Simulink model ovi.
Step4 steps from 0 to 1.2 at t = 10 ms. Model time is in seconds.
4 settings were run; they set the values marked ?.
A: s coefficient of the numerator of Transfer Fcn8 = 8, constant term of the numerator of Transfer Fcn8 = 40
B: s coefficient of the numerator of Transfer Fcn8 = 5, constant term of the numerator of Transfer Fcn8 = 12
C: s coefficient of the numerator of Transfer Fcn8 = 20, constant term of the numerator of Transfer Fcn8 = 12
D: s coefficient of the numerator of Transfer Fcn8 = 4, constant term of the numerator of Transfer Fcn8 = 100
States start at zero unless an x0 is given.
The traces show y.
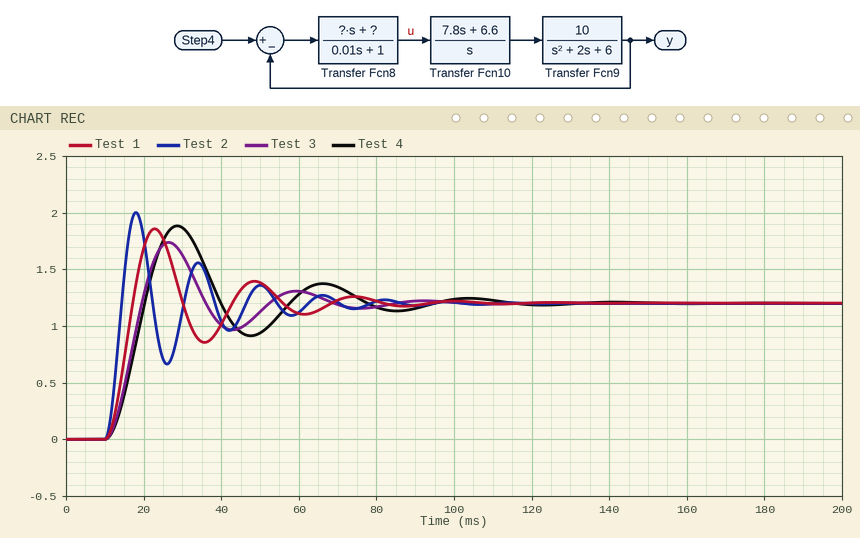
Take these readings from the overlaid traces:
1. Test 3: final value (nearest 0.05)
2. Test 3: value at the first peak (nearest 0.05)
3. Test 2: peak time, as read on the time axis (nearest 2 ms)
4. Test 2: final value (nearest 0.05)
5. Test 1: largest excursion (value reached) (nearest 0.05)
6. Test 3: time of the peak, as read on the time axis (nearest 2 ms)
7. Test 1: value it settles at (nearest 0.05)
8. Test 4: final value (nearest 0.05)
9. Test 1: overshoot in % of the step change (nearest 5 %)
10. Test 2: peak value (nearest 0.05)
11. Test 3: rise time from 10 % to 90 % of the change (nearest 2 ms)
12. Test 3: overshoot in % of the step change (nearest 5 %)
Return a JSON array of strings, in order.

["1.20", "1.75", "18 ms", "1.20", "1.85", "26 ms", "1.20", "1.20", "55 %", "2.00", "6 ms", "45 %"]
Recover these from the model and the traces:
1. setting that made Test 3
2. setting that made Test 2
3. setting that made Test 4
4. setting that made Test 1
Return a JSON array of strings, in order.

["B", "C", "D", "A"]
